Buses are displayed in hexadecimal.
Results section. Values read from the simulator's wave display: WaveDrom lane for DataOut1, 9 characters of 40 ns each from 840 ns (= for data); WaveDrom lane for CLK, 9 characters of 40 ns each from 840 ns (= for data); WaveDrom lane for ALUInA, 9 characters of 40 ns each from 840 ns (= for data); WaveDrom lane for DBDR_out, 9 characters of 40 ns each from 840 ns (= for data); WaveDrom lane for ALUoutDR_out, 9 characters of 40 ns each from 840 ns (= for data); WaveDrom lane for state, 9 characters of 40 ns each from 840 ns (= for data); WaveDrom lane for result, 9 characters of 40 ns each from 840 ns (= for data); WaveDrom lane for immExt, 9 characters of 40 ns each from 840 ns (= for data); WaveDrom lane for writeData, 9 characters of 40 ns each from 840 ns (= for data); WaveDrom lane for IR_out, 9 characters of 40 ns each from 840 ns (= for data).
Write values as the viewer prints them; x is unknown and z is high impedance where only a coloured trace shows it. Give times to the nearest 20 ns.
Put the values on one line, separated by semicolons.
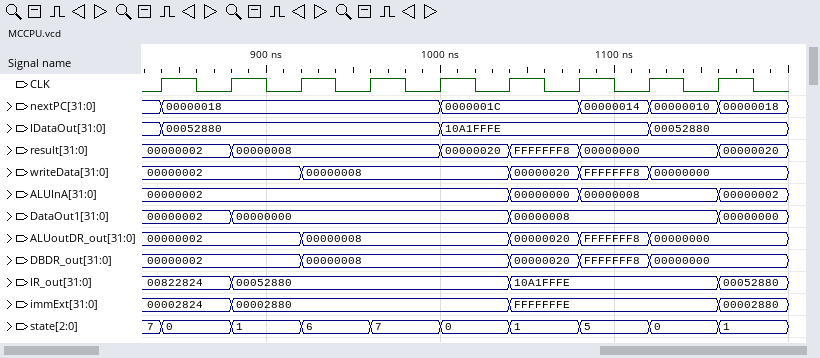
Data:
{name: 'DataOut1', wave: '==...=..=', data: '00000002 00000000 00000008 00000000'}; {name: 'CLK', wave: 'p........'}; {name: 'ALUInA', wave: '=....==.=', data: '00000002 00000000 00000008 00000002'}; {name: 'DBDR_out', wave: '=.=..===.', data: '00000002 00000008 00000020 FFFFFFF8 00000000'}; {name: 'ALUoutDR_out', wave: '=.=..===.', data: '00000002 00000008 00000020 FFFFFFF8 00000000'}; {name: 'state', wave: '=========', data: '0 1 6 7 0 1 5 0 1'}; {name: 'result', wave: '==..===.=', data: '00000002 00000008 00000020 FFFFFFF8 00000000 00000020'}; {name: 'immExt', wave: '==...=..=', data: '00002824 00002880 FFFFFFFE 00002880'}; {name: 'writeData', wave: '=.=..===.', data: '00000002 00000008 00000020 FFFFFFF8 00000000'}; {name: 'IR_out', wave: '==...=..=', data: '00822824 00052880 10A1FFFE 00052880'}
